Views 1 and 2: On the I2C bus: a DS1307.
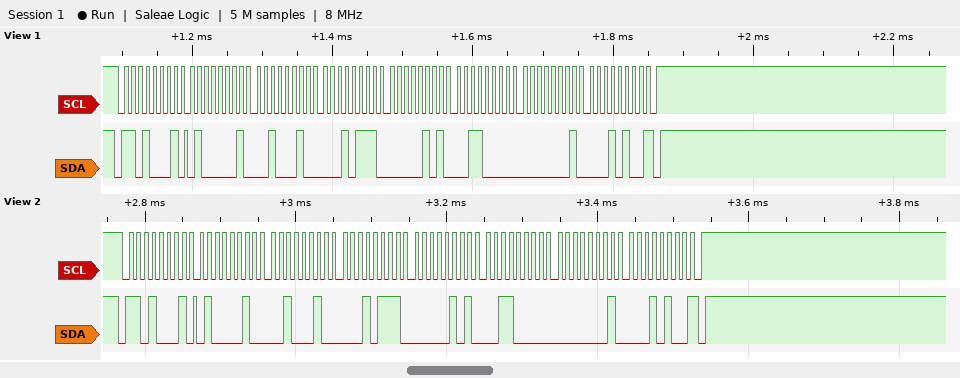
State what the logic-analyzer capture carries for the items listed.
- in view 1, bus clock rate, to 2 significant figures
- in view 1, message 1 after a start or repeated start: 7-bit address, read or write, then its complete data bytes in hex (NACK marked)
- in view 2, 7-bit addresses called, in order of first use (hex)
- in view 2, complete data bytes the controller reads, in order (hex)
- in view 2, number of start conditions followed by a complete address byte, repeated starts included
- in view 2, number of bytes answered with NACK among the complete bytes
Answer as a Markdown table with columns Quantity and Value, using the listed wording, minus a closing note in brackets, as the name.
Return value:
| Quantity | Value |
|---|---|
| in view 1, bus clock rate, to 2 significant figures | 100 kHz |
| in view 1, message 1 after a start or repeated start: 7-bit address, read or write, then its complete data bytes in hex | 0x68 read: 41 22 17 05 30 01 14 NACK |
| in view 2, 7-bit addresses called, in order of first use | 0x68 |
| in view 2, complete data bytes the controller reads, in order | 42 22 17 05 30 01 14 |
| in view 2, number of start conditions followed by a complete address byte, repeated starts included | 1 |
| in view 2, number of bytes answered with NACK among the complete bytes | 1 |
